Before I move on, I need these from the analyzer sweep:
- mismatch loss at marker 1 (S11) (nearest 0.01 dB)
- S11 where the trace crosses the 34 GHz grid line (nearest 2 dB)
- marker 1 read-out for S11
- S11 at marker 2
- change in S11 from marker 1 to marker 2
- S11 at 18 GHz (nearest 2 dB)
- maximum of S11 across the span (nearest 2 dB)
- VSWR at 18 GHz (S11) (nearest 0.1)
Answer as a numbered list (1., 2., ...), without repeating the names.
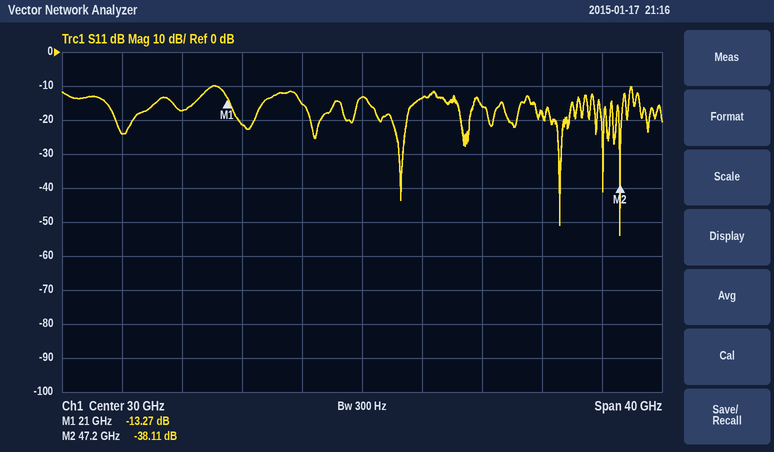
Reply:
1. 0.21 dB
2. -14 dB
3. -13.27 dB
4. -38.11 dB
5. -24.84 dB
6. -18 dB
7. -10 dB
8. 1.3
